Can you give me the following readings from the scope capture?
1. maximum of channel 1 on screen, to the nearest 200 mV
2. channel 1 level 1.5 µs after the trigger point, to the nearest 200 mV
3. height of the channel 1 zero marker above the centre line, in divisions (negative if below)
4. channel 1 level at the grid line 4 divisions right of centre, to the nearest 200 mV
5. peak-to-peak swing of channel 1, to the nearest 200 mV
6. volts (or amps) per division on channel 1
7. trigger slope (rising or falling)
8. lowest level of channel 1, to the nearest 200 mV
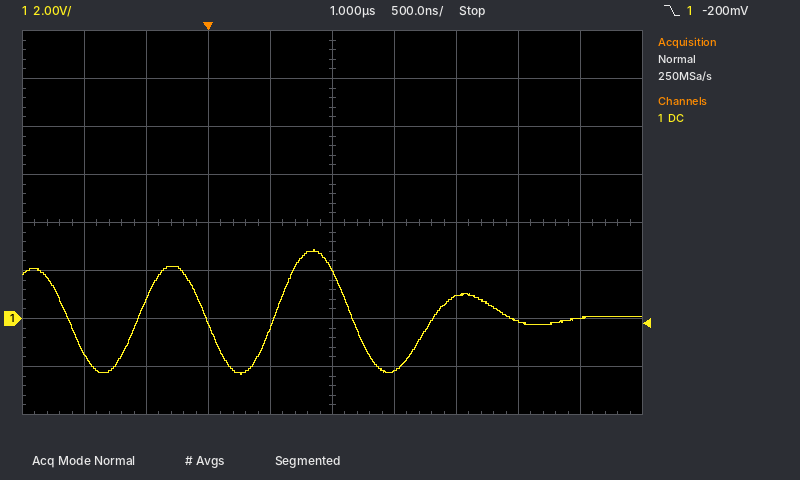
2.8 V
-2.2 V
-2.0 div
0.0 V
5.2 V
2 V
falling
-2.4 V
